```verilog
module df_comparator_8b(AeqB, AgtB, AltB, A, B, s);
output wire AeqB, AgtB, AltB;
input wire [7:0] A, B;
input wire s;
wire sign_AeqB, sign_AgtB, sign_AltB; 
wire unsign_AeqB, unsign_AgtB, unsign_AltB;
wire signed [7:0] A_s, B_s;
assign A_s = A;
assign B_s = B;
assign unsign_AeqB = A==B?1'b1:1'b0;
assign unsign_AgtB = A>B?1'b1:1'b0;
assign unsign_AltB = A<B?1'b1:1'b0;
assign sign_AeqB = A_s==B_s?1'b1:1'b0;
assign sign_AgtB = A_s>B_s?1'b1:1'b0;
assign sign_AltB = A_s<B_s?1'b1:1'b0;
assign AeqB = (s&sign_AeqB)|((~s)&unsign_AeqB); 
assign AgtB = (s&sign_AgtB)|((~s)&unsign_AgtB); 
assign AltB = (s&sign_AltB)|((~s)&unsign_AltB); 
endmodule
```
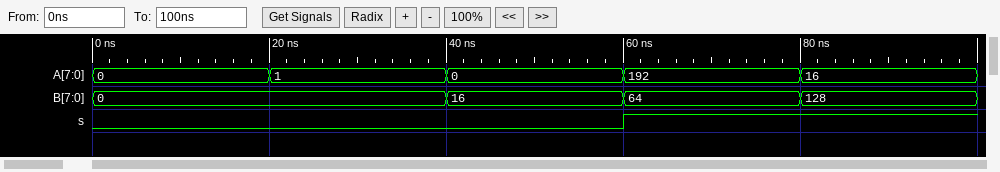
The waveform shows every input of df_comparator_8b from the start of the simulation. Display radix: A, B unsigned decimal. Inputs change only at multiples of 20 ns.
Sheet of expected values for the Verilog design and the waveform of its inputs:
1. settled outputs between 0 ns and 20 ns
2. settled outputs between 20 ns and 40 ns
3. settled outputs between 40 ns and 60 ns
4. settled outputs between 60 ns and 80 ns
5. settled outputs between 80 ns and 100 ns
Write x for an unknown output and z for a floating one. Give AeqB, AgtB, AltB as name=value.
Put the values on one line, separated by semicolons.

AeqB=1, AgtB=0, AltB=0; AeqB=0, AgtB=1, AltB=0; AeqB=0, AgtB=0, AltB=1; AeqB=0, AgtB=0, AltB=1; AeqB=0, AgtB=1, AltB=0
